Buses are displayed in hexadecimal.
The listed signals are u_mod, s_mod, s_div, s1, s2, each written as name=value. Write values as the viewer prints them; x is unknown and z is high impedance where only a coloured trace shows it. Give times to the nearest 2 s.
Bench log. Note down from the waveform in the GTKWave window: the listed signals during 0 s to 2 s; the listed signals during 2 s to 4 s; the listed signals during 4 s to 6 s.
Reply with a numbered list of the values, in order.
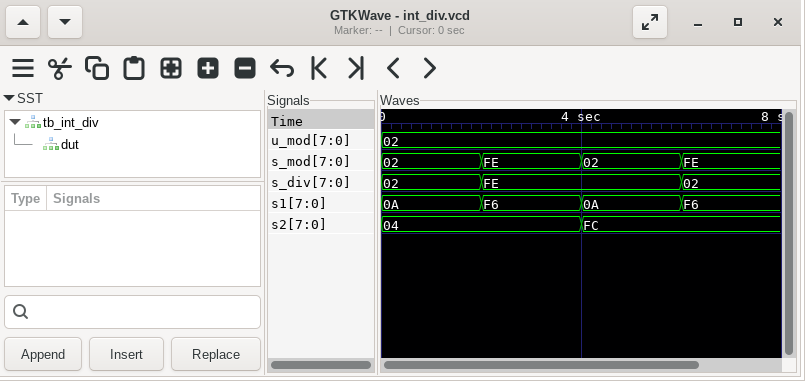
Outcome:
1. u_mod=02, s_mod=02, s_div=02, s1=0A, s2=04
2. u_mod=02, s_mod=FE, s_div=FE, s1=F6, s2=04
3. u_mod=02, s_mod=02, s_div=FE, s1=0A, s2=FC
